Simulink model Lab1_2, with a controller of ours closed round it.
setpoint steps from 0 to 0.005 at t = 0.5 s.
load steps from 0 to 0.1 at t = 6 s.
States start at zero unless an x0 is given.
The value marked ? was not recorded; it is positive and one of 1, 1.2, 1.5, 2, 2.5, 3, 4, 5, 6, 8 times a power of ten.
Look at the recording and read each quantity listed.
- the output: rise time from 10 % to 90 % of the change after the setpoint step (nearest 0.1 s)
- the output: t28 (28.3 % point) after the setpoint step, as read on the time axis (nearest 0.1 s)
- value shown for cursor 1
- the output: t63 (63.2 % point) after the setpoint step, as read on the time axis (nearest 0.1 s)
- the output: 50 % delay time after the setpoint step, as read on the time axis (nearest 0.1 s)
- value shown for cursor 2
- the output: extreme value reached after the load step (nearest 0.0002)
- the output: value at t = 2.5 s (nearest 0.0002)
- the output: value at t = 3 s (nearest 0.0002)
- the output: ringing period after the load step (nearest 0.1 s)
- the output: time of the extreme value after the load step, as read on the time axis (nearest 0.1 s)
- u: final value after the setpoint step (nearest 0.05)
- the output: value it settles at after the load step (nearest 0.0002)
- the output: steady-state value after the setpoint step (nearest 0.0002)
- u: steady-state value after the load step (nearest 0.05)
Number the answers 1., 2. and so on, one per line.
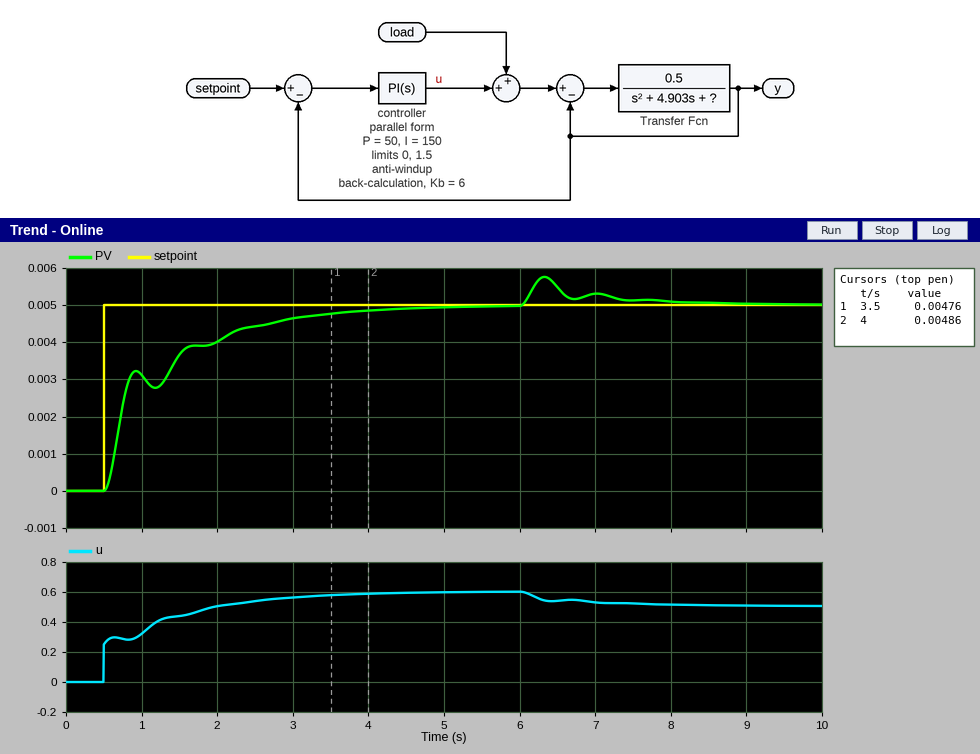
1. 2.1 s
2. 0.7 s
3. 0.00476
4. 0.9 s
5. 0.8 s
6. 0.00486
7. 0.0058
8. 0.0044
9. 0.0046
10. 0.7 s
11. 6.3 s
12. 0.60
13. 0.0050
14. 0.0050
15. 0.50
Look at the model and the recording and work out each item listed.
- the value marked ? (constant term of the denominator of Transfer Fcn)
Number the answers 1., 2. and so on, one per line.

1. 60
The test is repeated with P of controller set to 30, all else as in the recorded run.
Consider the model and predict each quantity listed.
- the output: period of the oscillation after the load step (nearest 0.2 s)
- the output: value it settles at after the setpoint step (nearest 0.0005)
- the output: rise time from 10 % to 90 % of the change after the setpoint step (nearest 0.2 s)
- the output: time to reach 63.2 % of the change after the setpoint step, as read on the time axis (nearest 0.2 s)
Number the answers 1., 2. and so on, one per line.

1. 0.8 s
2. 0.0050
3. 1.8 s
4. 1.4 s
